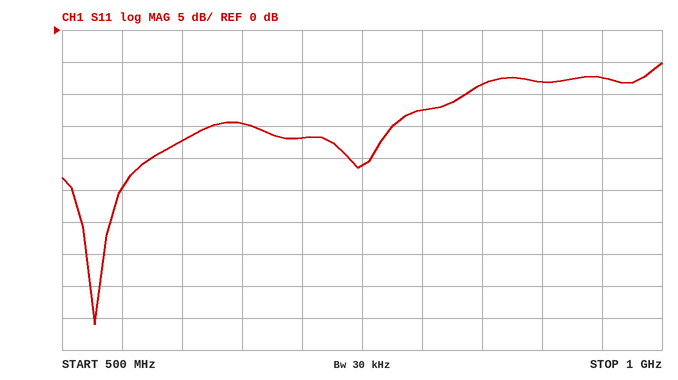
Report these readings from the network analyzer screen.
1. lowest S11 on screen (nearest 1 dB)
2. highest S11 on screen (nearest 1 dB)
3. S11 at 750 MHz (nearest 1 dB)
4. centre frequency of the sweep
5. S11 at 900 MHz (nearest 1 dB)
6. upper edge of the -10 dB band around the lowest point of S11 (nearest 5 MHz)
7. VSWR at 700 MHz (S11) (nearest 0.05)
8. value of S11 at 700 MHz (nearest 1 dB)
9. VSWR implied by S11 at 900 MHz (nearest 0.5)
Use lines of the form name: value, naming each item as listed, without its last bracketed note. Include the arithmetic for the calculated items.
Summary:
lowest S11 on screen: -46 dB
highest S11 on screen: -5 dB
S11 at 750 MHz: -21 dB
centre frequency of the sweep: 750 MHz
S11 at 900 MHz: -8 dB
upper edge of the -10 dB band around the lowest point of S11: 835 MHz
VSWR at 700 MHz (S11): |Γ| = 10^(-17/20) = 0.1413; VSWR = (1 + 0.1413)/(1 − 0.1413) ≈ 1.33, so 1.35 to the nearest 0.05
value of S11 at 700 MHz: -17 dB
VSWR implied by S11 at 900 MHz: |Γ| = 10^(-8/20) = 0.3981; VSWR = (1 + 0.3981)/(1 − 0.3981) ≈ 2.32, so 2.5 to the nearest 0.5
